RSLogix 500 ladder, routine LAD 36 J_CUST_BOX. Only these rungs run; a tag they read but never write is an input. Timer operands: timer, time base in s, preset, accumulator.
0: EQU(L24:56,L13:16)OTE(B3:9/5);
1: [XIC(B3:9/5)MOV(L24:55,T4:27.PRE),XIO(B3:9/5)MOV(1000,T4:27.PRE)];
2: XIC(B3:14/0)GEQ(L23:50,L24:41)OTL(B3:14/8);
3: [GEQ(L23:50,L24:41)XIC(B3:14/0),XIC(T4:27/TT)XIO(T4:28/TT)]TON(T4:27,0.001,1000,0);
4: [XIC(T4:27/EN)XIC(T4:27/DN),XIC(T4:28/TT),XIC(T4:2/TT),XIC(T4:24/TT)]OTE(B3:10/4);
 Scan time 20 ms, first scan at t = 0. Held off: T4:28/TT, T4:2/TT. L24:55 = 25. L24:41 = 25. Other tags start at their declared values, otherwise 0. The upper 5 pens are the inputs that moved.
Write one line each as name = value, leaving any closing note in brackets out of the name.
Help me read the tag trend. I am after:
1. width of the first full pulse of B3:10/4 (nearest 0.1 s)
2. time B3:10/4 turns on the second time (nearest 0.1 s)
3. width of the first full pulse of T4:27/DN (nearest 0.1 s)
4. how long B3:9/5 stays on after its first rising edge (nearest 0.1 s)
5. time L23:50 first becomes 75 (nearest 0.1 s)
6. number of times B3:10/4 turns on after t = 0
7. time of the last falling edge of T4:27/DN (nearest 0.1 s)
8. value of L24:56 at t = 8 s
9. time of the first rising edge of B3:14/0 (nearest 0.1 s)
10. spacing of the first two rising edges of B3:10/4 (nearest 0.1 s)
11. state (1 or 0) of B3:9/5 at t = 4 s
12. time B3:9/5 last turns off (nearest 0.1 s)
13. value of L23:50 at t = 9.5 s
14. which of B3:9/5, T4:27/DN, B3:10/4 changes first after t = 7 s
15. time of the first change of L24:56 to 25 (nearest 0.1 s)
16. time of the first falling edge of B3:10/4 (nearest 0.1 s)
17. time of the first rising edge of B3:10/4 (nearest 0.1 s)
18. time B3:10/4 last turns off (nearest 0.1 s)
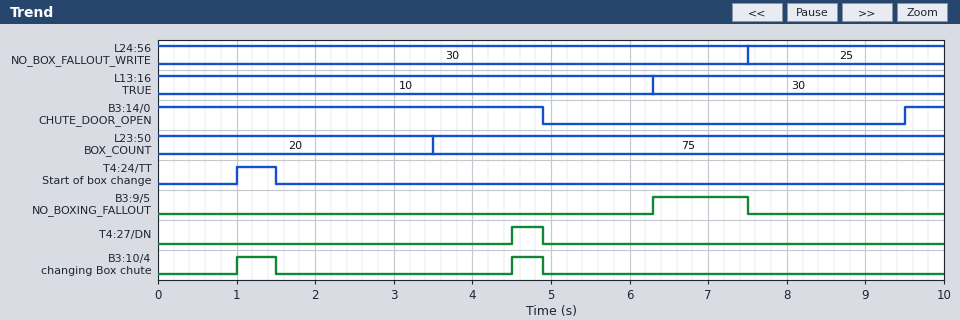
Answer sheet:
width of the first full pulse of B3:10/4 = 0.5 s
time B3:10/4 turns on the second time = 4.5 s
width of the first full pulse of T4:27/DN = 0.4 s
how long B3:9/5 stays on after its first rising edge = 1.2 s
time L23:50 first becomes 75 = 3.5 s
number of times B3:10/4 turns on after t = 0 = 2
time of the last falling edge of T4:27/DN = 4.9 s
value of L24:56 at t = 8 s = 25
time of the first rising edge of B3:14/0 = 9.5 s
spacing of the first two rising edges of B3:10/4 = 3.5 s
state (1 or 0) of B3:9/5 at t = 4 s = 0
time B3:9/5 last turns off = 7.5 s
value of L23:50 at t = 9.5 s = 75
which of B3:9/5, T4:27/DN, B3:10/4 changes first after t = 7 s = B3:9/5
time of the first change of L24:56 to 25 = 7.5 s
time of the first falling edge of B3:10/4 = 1.5 s
time of the first rising edge of B3:10/4 = 1.0 s
time B3:10/4 last turns off = 4.9 s
